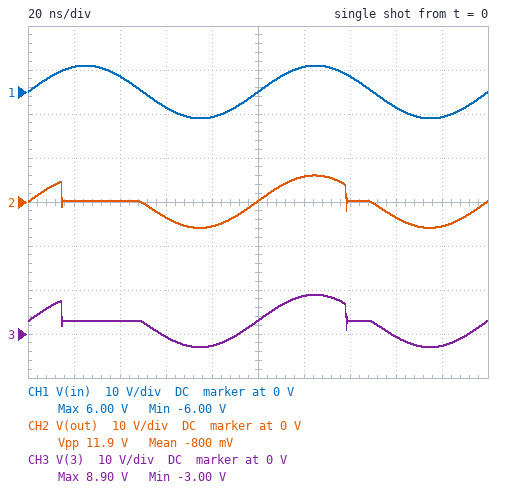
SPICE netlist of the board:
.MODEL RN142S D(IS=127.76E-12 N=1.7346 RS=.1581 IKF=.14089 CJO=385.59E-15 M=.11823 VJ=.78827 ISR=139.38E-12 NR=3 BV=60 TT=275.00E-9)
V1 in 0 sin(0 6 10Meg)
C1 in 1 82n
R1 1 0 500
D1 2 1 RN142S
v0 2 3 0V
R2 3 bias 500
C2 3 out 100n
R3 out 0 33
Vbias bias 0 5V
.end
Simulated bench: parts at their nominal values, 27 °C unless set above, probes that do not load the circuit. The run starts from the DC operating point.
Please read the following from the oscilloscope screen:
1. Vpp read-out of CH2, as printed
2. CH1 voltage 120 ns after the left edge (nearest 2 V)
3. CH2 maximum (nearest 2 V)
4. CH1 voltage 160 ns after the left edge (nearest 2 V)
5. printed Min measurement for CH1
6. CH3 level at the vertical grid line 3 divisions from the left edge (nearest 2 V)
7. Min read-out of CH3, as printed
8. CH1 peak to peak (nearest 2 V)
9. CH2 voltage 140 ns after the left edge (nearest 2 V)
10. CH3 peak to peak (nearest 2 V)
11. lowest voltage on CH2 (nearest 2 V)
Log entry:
11.9 V
6 V
6 V
-4 V
-6.00 V
0 V
-3.00 V
12 V
0 V
12 V
-6 V
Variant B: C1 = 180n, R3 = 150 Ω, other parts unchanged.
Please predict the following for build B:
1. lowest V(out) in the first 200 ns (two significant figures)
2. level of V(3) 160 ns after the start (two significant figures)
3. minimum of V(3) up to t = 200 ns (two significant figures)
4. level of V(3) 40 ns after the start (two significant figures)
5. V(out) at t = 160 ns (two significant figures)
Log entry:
-6.0 V
-700 mV
-3.1 V
3.4 V
-3.6 V
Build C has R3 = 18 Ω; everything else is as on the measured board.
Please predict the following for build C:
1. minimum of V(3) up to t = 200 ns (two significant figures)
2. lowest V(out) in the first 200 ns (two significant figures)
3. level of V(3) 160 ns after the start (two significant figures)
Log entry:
-2.9 V
-5.8 V
-600 mV
